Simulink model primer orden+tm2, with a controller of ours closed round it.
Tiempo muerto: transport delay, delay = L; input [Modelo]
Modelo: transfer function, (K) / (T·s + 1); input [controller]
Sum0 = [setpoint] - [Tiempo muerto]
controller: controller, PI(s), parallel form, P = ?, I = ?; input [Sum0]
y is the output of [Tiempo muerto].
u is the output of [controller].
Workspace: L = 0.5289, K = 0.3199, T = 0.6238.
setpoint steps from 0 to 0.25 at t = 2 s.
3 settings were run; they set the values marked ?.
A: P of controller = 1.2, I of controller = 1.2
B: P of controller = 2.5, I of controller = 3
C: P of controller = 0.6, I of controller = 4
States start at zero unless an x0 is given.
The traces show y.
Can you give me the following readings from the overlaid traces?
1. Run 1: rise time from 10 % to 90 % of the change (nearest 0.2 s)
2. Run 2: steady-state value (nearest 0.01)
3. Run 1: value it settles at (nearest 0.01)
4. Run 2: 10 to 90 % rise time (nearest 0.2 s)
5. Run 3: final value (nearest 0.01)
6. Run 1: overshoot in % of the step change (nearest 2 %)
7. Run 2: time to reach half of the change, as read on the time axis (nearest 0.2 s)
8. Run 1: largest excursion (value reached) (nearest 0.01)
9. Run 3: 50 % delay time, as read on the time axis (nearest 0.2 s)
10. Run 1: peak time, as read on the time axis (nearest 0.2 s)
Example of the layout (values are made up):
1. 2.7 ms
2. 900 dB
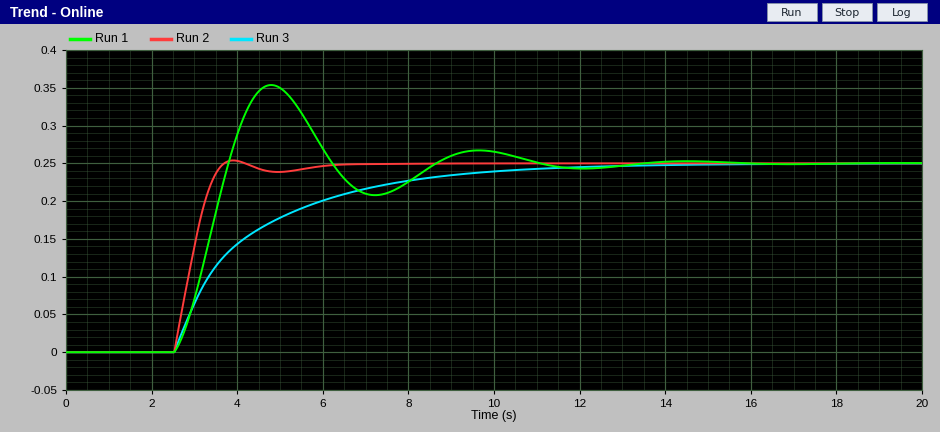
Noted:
1. 1.0 s
2. 0.25
3. 0.25
4. 0.8 s
5. 0.25
6. 42 %
7. 3.0 s
8. 0.35
9. 3.6 s
10. 4.8 s
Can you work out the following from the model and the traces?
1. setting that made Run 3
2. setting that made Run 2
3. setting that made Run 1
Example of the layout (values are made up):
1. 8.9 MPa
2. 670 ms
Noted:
1. A
2. B
3. C
